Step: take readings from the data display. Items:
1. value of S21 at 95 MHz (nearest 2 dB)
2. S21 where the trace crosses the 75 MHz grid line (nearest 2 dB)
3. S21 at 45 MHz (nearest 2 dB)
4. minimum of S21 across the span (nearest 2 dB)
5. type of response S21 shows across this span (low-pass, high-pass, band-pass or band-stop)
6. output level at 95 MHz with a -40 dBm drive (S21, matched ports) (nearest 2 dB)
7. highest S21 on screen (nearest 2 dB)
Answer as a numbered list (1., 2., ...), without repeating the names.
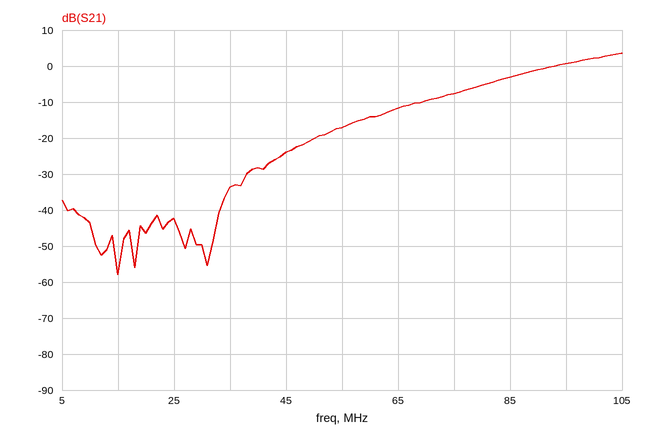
1. 0 dB
2. -8 dB
3. -24 dB
4. -58 dB
5. high-pass
6. -40 dBm
7. 4 dB
